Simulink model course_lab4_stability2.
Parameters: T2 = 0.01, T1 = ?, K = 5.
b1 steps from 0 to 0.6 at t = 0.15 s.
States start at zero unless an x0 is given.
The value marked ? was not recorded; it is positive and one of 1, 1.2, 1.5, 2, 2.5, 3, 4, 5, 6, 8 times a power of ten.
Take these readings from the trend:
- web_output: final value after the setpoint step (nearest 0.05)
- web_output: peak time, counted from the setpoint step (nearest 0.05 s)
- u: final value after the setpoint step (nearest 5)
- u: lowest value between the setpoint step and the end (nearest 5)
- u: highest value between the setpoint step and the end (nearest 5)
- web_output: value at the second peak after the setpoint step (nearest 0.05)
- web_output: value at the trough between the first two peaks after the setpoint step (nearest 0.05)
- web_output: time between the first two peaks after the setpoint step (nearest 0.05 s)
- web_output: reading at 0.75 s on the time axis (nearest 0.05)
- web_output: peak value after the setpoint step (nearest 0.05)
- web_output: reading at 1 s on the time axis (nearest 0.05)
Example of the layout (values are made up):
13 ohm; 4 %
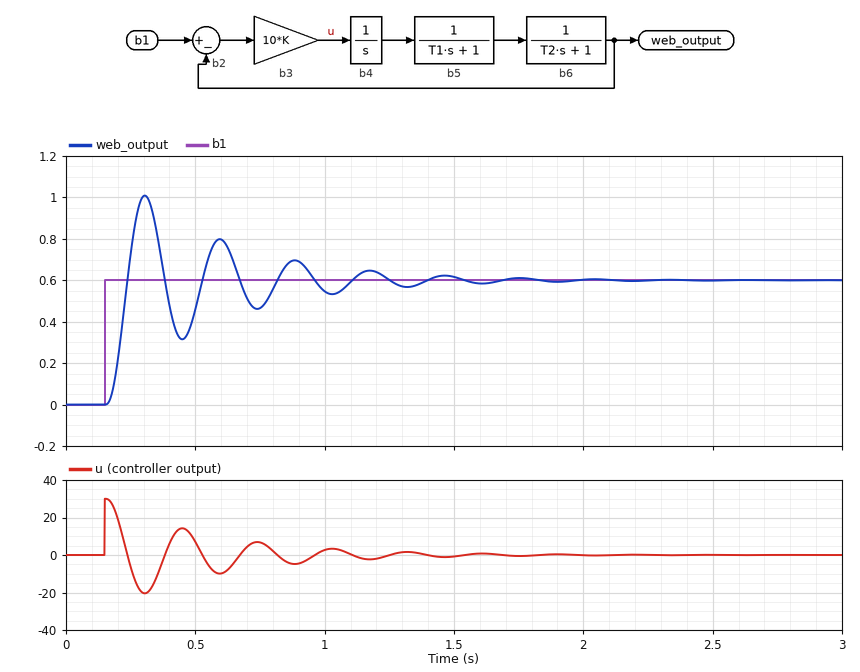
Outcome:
0.60; 0.15 s; 0; -20; 30; 0.80; 0.30; 0.30 s; 0.45; 1.00; 0.55
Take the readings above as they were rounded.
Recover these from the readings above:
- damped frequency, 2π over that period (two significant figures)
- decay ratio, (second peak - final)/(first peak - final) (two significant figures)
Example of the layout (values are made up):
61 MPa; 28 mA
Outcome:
21 rad/s; 0.50
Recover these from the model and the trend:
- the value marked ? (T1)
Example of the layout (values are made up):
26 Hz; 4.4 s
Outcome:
0.1
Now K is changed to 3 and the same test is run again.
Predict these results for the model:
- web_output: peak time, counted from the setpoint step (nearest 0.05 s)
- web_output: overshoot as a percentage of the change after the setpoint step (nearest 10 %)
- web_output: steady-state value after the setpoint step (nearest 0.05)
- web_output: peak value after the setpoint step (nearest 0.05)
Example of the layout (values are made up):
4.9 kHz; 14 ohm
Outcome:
0.20 s; 50 %; 0.60; 0.90
